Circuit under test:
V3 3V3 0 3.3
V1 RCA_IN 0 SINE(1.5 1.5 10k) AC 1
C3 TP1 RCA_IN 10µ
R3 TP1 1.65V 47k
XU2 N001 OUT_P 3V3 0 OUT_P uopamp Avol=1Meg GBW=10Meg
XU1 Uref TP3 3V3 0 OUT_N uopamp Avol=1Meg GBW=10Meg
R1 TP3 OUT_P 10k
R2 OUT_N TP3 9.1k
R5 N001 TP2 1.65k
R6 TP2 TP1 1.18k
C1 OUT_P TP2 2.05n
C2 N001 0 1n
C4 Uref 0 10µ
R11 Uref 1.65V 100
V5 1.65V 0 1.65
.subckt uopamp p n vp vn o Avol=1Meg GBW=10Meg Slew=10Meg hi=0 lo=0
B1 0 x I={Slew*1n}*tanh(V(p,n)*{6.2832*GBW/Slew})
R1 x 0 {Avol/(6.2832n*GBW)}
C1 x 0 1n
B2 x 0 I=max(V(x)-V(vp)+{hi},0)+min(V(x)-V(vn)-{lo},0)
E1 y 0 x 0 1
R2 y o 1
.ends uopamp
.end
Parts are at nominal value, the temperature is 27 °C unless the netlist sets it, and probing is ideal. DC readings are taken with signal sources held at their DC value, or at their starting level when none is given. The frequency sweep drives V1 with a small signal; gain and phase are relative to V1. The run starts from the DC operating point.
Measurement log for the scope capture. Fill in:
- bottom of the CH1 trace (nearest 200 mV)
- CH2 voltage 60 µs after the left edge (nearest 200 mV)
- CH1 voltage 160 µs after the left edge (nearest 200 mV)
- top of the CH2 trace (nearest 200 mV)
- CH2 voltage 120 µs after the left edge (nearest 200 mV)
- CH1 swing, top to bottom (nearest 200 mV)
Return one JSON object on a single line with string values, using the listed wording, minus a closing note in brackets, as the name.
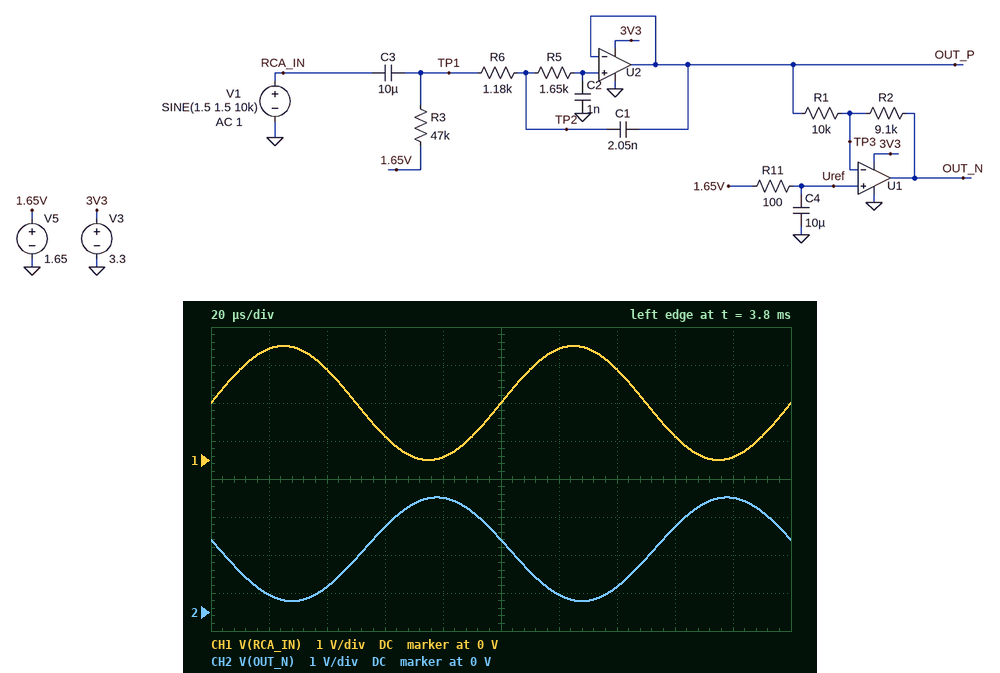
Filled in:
{"bottom of the CH1 trace": "0 V", "CH2 voltage 60 µs after the left edge": "2.2 V", "CH1 voltage 160 µs after the left edge": "600 mV", "top of the CH2 trace": "3.0 V", "CH2 voltage 120 µs after the left edge": "400 mV", "CH1 swing, top to bottom": "3.0 V"}
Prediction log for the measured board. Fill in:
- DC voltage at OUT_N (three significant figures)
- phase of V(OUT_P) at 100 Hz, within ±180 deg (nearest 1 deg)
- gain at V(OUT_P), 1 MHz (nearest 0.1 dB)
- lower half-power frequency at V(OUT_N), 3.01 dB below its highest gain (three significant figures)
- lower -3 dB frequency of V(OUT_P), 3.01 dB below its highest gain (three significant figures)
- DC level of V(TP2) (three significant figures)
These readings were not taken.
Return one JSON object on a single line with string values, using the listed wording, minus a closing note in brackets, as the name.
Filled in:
{"DC voltage at OUT_N": "1.65 V", "phase of V(OUT_P) at 100 Hz, within ±180 deg": "0 deg", "gain at V(OUT_P), 1 MHz": "-44.1 dB", "lower half-power frequency at V(OUT_N), 3.01 dB below its highest gain": "339 mHz", "lower -3 dB frequency of V(OUT_P), 3.01 dB below its highest gain": "339 mHz", "DC level of V(TP2)": "1.65 V"}
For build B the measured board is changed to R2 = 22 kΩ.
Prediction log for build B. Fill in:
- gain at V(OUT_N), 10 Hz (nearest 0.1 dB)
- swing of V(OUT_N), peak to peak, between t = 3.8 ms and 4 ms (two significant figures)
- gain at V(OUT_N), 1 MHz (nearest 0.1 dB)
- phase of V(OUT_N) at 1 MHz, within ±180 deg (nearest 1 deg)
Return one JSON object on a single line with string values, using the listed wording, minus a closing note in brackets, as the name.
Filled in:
{"gain at V(OUT_N), 10 Hz": "6.8 dB", "swing of V(OUT_N), peak to peak, between t = 3.8 ms and 4 ms": "3.3 V", "gain at V(OUT_N), 1 MHz": "-37.7 dB", "phase of V(OUT_N) at 1 MHz, within ±180 deg": "-18 deg"}
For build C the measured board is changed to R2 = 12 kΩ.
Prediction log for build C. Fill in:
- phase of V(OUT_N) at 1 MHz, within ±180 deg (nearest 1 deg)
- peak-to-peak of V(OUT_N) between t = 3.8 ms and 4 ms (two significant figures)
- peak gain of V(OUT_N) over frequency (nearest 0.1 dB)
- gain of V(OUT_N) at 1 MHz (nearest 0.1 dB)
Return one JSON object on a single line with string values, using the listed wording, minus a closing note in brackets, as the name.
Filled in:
{"phase of V(OUT_N) at 1 MHz, within ±180 deg": "-12 deg", "peak-to-peak of V(OUT_N) between t = 3.8 ms and 4 ms": "3.3 V", "peak gain of V(OUT_N) over frequency": "1.6 dB", "gain of V(OUT_N) at 1 MHz": "-42.7 dB"}
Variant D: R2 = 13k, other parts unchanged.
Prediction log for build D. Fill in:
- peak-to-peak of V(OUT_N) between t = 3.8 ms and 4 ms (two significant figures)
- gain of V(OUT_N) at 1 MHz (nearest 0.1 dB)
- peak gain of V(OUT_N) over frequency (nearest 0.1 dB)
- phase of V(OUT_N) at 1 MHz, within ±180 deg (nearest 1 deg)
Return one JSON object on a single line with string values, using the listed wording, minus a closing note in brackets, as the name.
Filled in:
{"peak-to-peak of V(OUT_N) between t = 3.8 ms and 4 ms": "3.3 V", "gain of V(OUT_N) at 1 MHz": "-42.0 dB", "peak gain of V(OUT_N) over frequency": "2.3 dB", "phase of V(OUT_N) at 1 MHz, within ±180 deg": "-13 deg"}
